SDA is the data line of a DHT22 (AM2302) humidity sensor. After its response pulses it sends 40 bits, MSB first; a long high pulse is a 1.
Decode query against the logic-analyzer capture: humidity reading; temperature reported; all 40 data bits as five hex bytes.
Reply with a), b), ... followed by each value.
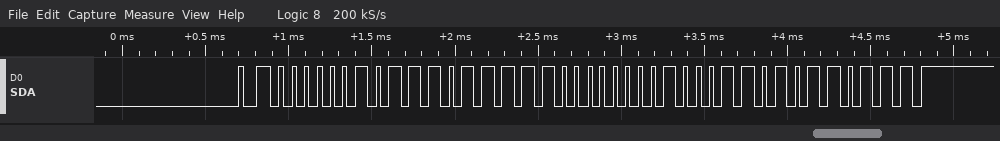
a) 75.1 %
b) -7.0 °C
c) 02 EF 80 46 B7
